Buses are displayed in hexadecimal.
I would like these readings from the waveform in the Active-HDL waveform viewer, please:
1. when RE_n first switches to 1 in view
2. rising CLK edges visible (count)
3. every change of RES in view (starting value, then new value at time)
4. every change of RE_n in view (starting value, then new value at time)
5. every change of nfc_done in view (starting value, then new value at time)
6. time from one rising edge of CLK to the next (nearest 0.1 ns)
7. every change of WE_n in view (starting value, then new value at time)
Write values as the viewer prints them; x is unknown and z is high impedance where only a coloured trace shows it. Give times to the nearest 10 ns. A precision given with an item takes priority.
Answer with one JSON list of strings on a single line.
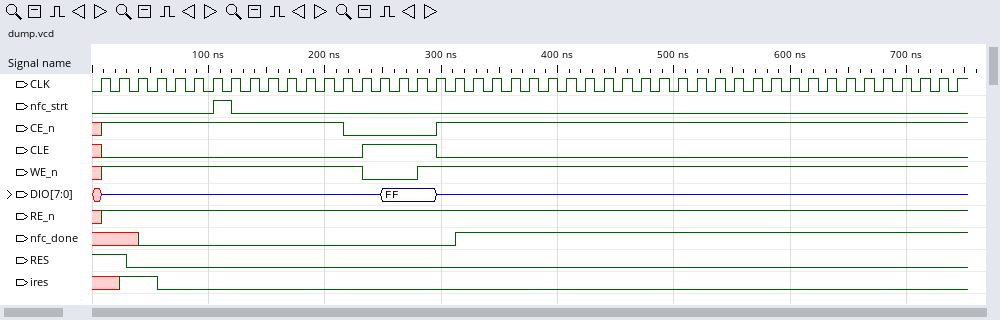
["10 ns", "47", "1, 0 at 30 ns", "x, 1 at 10 ns", "x, 0 at 40 ns, 1 at 310 ns", "16 ns", "x, 1 at 10 ns, 0 at 230 ns, 1 at 280 ns"]
